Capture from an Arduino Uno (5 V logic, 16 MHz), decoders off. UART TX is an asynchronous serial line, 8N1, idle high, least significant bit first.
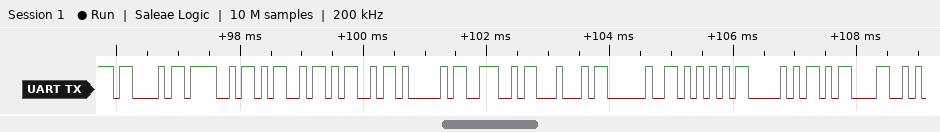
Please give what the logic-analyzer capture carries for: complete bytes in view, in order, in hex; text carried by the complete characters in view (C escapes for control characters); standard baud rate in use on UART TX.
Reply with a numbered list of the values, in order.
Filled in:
1. 0x43 0x4F 0x4D 0x4D 0x41 0x4E 0x44 0x20 0x55 0x50 0x0D
2. "COMMAND UP\r"
3. 9600 baud
